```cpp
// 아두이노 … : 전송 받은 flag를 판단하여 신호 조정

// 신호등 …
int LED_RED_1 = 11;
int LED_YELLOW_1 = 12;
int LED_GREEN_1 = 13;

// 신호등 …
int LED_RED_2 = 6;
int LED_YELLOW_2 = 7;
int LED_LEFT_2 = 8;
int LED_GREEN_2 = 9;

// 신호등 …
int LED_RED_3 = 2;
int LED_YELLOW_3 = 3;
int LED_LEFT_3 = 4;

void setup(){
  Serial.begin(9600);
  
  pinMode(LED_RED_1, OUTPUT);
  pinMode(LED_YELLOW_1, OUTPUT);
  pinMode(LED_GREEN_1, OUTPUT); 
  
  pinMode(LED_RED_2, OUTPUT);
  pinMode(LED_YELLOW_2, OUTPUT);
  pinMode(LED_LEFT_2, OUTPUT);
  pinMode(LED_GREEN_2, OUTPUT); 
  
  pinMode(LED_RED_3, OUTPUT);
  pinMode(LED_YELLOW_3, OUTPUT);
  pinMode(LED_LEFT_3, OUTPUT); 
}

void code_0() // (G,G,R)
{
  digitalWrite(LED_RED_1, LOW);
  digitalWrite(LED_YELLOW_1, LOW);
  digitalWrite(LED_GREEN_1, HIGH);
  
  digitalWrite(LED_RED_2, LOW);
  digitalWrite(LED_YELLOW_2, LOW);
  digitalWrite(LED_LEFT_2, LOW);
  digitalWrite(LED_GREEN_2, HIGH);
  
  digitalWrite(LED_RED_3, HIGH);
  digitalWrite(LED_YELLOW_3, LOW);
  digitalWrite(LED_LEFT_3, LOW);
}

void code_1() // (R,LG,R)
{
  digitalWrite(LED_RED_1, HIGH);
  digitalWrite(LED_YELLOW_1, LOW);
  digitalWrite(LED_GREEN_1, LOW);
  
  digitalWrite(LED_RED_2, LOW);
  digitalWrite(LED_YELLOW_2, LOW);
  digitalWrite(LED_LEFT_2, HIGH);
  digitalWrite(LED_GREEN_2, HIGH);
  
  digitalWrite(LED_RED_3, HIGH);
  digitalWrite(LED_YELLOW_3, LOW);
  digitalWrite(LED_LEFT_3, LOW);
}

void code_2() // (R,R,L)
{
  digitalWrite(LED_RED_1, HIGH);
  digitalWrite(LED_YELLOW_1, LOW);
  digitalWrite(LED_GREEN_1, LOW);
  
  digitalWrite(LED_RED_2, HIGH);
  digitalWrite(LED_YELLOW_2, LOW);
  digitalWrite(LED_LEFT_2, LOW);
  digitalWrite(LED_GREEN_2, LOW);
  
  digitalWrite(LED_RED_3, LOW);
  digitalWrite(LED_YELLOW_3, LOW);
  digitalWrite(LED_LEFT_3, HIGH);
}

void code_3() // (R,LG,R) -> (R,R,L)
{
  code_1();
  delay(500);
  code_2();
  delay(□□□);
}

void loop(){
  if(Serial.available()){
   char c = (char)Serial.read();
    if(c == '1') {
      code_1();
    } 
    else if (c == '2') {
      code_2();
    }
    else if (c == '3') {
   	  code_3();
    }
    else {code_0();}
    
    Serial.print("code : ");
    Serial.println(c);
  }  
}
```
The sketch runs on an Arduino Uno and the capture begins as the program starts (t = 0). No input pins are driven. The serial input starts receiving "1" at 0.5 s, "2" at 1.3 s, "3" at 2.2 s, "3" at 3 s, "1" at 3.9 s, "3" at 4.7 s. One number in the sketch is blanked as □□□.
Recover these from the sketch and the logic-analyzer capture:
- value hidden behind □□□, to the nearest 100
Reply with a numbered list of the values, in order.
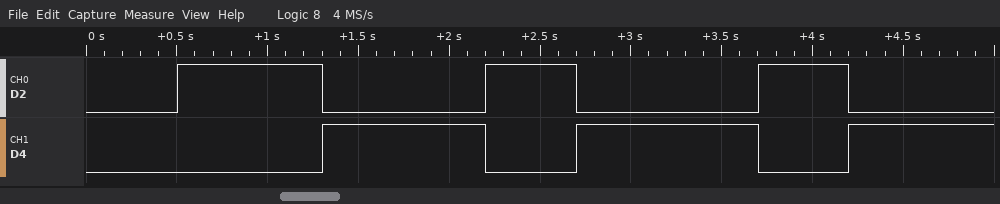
1. 1000
